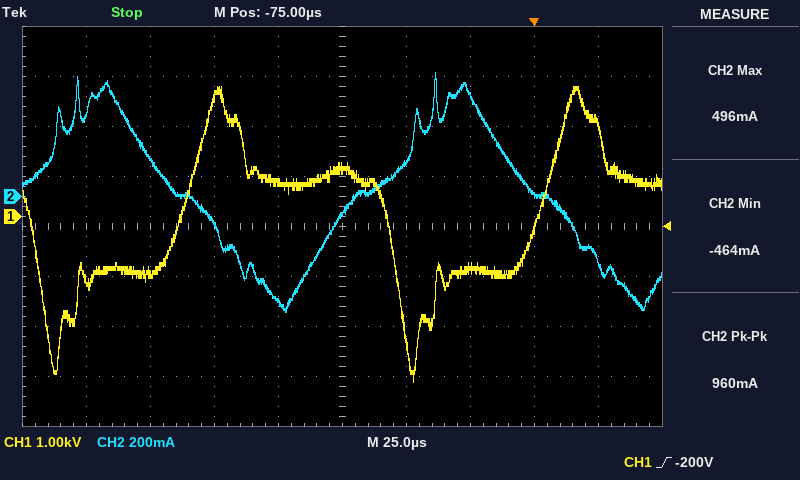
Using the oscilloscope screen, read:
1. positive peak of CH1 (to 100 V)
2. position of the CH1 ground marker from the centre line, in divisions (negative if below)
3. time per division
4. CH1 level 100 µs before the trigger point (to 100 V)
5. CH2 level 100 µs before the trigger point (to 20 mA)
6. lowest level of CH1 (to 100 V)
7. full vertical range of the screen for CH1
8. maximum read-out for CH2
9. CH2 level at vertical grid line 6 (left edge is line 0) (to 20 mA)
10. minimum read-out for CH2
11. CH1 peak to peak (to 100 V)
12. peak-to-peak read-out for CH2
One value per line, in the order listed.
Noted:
2.6 kV
+0.2 div
25 µs
700 V
-420 mA
-3.3 kV
8 kV
496 mA
140 mA
-464 mA
5.9 kV
960 mA
